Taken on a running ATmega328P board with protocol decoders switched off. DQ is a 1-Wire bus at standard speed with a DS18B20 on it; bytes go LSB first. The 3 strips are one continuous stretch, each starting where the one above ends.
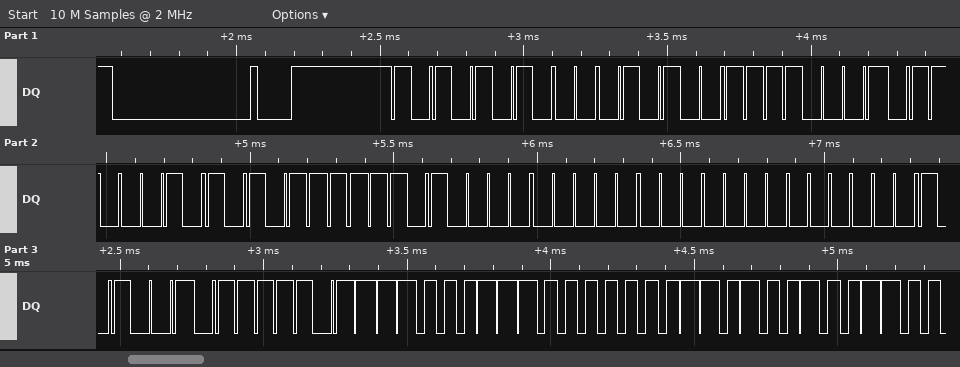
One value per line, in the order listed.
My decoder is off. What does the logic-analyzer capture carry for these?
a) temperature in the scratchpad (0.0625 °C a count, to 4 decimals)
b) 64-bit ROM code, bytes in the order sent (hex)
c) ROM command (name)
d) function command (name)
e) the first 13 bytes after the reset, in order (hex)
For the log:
28.4375 °C
28 8F 46 F5 0B 00 00 94
Match ROM
Read Scratchpad
55 28 8F 46 F5 0B 00 00 94 BE C7 01 4B
